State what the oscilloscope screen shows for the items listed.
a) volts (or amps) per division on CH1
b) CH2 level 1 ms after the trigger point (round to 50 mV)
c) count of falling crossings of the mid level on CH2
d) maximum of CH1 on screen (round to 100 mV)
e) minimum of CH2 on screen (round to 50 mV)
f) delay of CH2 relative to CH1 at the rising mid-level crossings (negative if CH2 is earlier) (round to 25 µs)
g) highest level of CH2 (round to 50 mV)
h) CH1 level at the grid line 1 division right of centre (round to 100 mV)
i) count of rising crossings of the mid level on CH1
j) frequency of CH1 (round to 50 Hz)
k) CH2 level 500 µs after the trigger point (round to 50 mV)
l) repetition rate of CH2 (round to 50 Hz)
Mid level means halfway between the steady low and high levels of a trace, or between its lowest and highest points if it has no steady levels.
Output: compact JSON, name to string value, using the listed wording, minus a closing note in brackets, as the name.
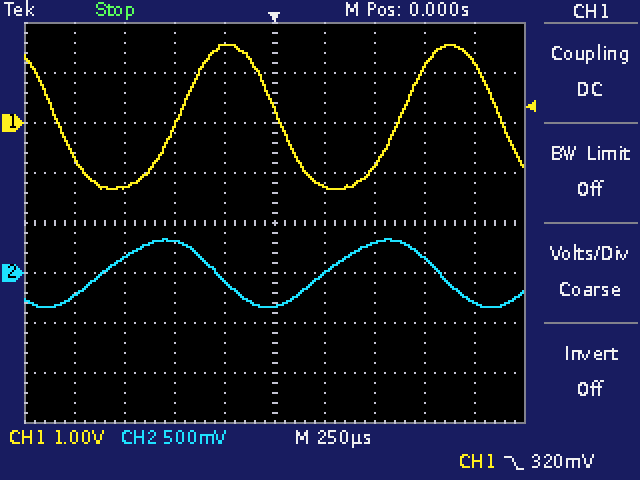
{"volts (or amps) per division on CH1": "1 V", "CH2 level 1 ms after the trigger point": "-300 mV", "count of falling crossings of the mid level on CH2": "2", "maximum of CH1 on screen": "1.6 V", "minimum of CH2 on screen": "-350 mV", "delay of CH2 relative to CH1 at the rising mid-level crossings (negative if CH2 is earlier)": "-375 µs", "highest level of CH2": "350 mV", "CH1 level at the grid line 1 division right of centre": "-1.3 V", "count of rising crossings of the mid level on CH1": "2", "frequency of CH1": "900 Hz", "CH2 level 500 µs after the trigger point": "300 mV", "repetition rate of CH2": "900 Hz"}
